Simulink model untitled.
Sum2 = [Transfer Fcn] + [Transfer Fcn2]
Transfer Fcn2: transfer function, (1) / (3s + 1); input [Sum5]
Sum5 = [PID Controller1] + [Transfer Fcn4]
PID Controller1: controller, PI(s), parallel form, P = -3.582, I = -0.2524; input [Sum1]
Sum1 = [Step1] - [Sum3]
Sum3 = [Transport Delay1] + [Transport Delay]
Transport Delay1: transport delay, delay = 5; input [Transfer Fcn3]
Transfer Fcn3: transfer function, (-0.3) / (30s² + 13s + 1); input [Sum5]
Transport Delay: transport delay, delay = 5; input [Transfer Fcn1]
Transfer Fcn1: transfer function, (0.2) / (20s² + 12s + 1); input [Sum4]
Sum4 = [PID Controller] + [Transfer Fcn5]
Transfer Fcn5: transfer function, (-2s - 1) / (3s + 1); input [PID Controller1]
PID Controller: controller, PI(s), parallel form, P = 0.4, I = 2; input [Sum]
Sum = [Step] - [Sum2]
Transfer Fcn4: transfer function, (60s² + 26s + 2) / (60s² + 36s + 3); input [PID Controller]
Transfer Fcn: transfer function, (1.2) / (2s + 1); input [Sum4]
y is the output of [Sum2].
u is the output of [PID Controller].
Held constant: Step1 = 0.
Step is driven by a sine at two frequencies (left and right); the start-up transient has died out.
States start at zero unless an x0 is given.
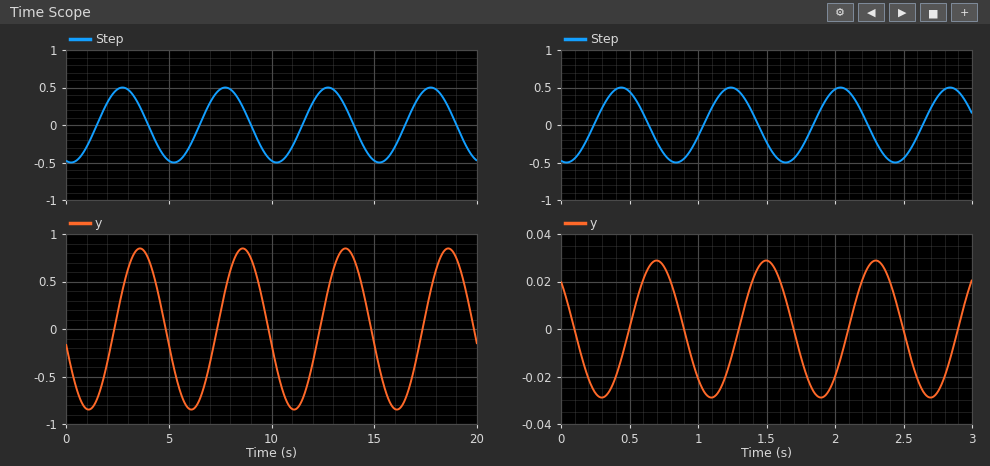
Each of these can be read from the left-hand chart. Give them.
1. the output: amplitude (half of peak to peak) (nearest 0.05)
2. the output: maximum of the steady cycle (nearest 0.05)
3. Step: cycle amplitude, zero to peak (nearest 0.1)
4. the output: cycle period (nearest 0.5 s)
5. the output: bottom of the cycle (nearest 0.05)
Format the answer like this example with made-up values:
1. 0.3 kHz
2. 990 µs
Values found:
1. 0.85
2. 0.85
3. 0.5
4. 5.0 s
5. -0.85
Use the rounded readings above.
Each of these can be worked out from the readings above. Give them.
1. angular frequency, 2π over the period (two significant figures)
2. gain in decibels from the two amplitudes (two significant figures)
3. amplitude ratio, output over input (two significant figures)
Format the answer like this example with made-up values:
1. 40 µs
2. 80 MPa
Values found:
1. 1.3 rad/s
2. 4.6 dB
3. 1.7
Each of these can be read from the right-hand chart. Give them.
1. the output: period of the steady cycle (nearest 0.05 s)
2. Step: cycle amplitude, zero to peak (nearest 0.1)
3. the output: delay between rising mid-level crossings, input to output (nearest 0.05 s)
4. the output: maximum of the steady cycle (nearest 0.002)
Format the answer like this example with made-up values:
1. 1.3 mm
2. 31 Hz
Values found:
1. 0.80 s
2. 0.5
3. 0.25 s
4. 0.028
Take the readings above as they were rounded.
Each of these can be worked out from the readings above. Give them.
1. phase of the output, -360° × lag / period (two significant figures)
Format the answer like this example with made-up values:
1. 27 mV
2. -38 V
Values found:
1. -110°
